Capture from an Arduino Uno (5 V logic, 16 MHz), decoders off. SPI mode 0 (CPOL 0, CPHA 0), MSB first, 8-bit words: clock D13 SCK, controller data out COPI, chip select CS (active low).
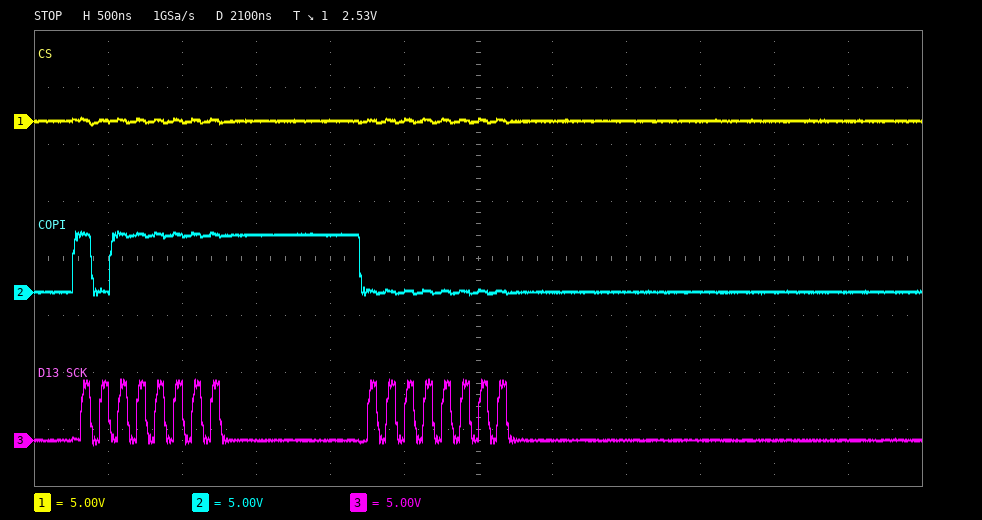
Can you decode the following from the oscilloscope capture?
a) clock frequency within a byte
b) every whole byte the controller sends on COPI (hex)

8 MHz
BF 00
